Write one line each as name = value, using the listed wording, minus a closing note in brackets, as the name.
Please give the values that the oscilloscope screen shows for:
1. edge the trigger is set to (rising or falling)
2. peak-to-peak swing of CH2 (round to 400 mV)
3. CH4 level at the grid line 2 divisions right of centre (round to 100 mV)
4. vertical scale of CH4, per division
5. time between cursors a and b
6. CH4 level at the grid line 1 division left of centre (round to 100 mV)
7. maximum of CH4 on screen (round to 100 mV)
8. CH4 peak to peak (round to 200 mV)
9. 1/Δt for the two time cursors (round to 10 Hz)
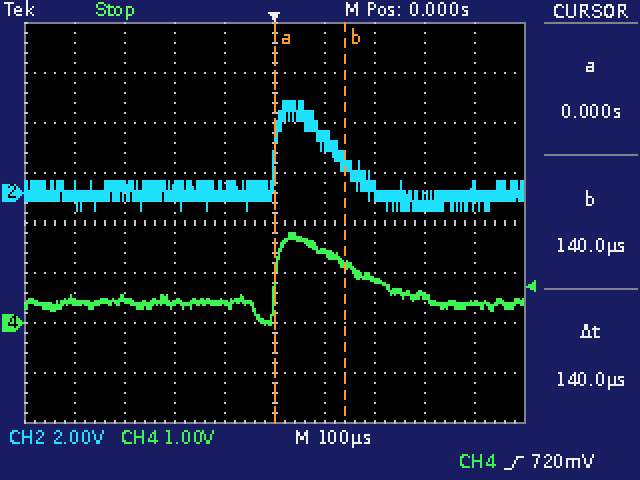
edge the trigger is set to = rising
peak-to-peak swing of CH2 = 4.4 V
CH4 level at the grid line 2 divisions right of centre = 900 mV
vertical scale of CH4, per division = 1 V
time between cursors a and b = 140 µs
CH4 level at the grid line 1 division left of centre = 400 mV
maximum of CH4 on screen = 1.8 V
CH4 peak to peak = 1.8 V
1/Δt for the two time cursors = 7.14 kHz
